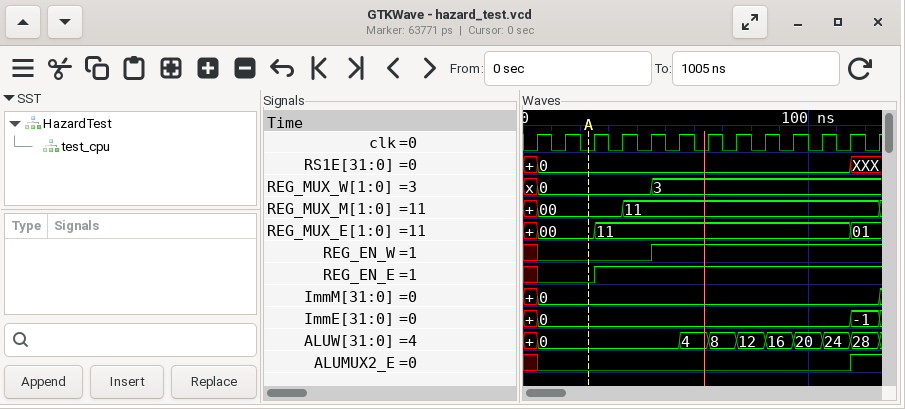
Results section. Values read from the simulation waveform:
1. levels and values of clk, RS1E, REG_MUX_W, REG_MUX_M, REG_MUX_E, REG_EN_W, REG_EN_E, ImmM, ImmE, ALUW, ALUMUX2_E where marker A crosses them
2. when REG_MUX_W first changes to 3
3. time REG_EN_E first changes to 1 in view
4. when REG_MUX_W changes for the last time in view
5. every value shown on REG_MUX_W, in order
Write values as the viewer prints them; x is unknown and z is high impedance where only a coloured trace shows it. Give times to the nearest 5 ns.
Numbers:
clk=0, RS1E=0, REG_MUX_W=0, REG_MUX_M=00, REG_MUX_E=00, REG_EN_W=0, REG_EN_E=0, ImmM=0, ImmE=0, ALUW=0, ALUMUX2_E=0
45 ns
25 ns
45 ns
x, 0, 3
